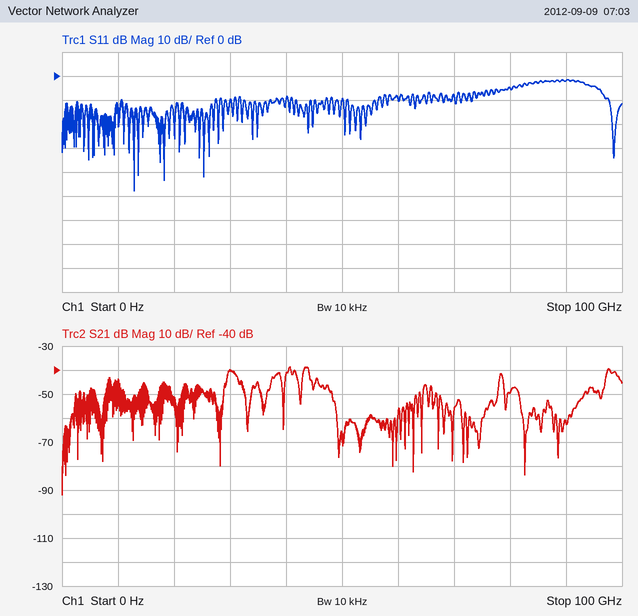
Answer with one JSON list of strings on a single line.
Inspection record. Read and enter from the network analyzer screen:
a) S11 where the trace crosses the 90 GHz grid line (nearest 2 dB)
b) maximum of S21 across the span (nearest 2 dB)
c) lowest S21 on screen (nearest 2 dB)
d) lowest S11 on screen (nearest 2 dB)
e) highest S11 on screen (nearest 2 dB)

["-2 dB", "-38 dB", "-92 dB", "-48 dB", "-2 dB"]
